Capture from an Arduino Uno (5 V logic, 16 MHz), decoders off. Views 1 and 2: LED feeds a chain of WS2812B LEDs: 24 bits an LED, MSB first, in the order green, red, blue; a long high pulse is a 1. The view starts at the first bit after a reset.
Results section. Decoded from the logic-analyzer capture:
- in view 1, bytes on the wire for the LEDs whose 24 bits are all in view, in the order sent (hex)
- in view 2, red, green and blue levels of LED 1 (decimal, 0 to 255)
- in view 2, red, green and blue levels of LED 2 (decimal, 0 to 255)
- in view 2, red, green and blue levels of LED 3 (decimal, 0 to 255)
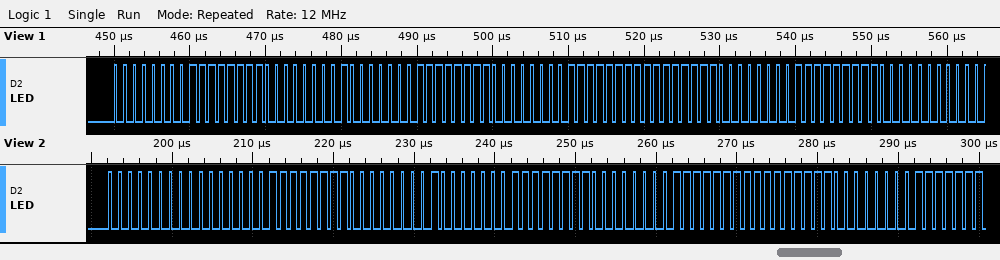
00 FF 00 80 FF 00 FF FF 00
0, 0, 255
128, 0, 255
255, 0, 255
